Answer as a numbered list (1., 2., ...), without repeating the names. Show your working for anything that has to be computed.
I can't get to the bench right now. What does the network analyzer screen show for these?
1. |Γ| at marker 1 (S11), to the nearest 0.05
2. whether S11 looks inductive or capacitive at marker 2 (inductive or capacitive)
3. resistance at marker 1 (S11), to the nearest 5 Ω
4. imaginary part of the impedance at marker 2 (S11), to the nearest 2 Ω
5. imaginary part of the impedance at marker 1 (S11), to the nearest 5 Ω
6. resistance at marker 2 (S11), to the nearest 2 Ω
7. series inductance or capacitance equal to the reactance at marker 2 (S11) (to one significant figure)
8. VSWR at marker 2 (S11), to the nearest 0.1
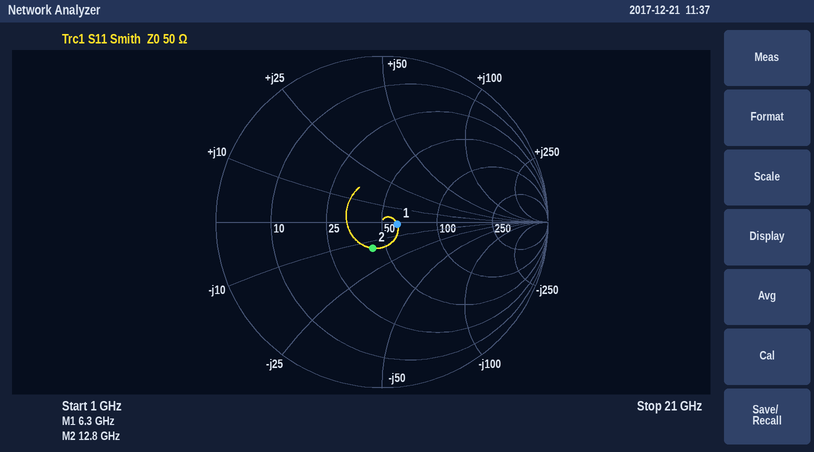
1. 0.10
2. capacitive
3. 60 Ω
4. -14 Ω
5. 0 Ω
6. 42 Ω
7. C = 1/(2π × 12.8 GHz × 14 Ω) ≈ 888 fF, so 900 fF to one significant figure
8. 1.4
